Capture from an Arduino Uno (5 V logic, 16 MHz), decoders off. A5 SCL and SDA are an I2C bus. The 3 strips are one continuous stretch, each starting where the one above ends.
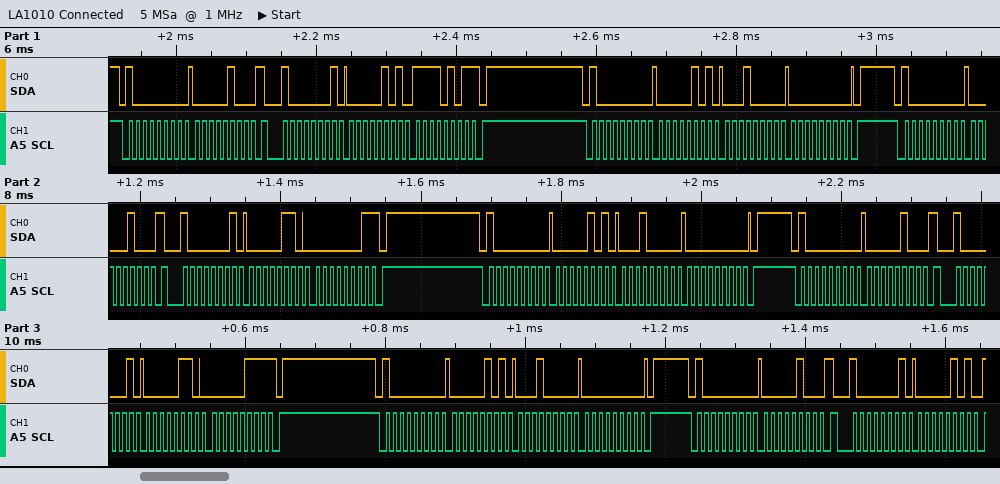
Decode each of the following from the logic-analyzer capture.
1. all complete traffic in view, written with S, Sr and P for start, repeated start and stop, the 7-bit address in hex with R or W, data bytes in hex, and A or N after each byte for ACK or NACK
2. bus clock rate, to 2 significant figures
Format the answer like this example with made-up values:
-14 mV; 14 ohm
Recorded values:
S 40W A 04 A Sr 40R A 05 A F5 N P S 40W A 05 A 10 A 00 A P S 40W A 04 A Sr 40R A 06 A 01 N P S 40W A 05 A 10 A 00 A P S 40W A 04 A Sr 40R A 06 A 07 N P S 40W A 05 A 10 A 00 A P S 40W A 04 A Sr 40R A 05 A; 100 kHz
